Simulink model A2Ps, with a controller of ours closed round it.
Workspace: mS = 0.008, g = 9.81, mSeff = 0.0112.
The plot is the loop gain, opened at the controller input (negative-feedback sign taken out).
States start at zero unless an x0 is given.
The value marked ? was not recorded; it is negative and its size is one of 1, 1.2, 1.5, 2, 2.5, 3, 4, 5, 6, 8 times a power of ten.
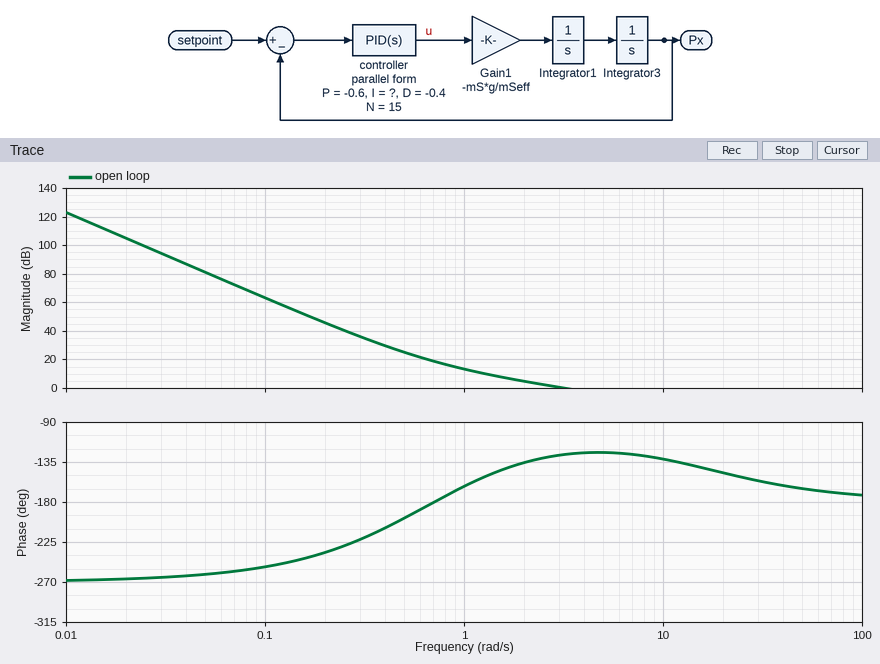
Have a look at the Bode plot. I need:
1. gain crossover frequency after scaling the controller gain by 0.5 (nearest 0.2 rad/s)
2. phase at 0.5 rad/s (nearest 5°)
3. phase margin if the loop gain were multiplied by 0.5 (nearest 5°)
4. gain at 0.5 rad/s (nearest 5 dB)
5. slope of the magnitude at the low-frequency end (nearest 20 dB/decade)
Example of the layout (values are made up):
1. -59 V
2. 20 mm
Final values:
1. 1.8 rad/s
2. -200°
3. 40°
4. 25 dB
5. -60 dB/decade
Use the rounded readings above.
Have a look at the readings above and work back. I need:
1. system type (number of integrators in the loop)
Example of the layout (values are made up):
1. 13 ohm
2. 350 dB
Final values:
1. 3
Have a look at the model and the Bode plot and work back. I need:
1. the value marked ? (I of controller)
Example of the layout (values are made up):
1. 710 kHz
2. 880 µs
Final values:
1. -0.2
